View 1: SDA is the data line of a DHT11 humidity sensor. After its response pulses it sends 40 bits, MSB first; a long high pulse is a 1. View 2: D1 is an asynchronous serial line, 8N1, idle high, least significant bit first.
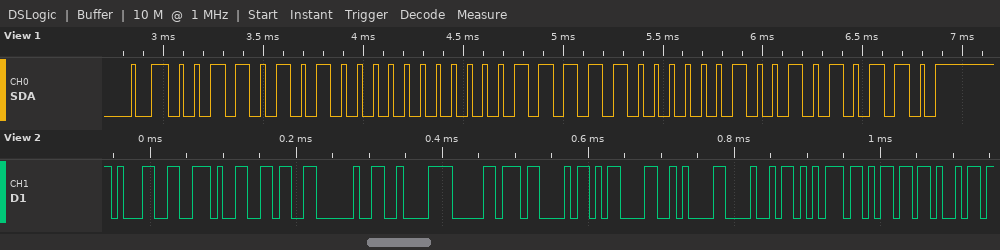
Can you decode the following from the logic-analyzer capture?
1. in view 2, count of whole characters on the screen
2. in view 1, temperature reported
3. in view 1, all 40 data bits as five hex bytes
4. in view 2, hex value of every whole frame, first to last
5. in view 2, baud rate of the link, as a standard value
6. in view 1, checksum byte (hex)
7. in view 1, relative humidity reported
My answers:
13
31.2 °C
35 00 1F 02 56
31 2E 36 20 C2 B0 43 0D 0A 48 75 6D 69
115200 baud
0x56
53 %
